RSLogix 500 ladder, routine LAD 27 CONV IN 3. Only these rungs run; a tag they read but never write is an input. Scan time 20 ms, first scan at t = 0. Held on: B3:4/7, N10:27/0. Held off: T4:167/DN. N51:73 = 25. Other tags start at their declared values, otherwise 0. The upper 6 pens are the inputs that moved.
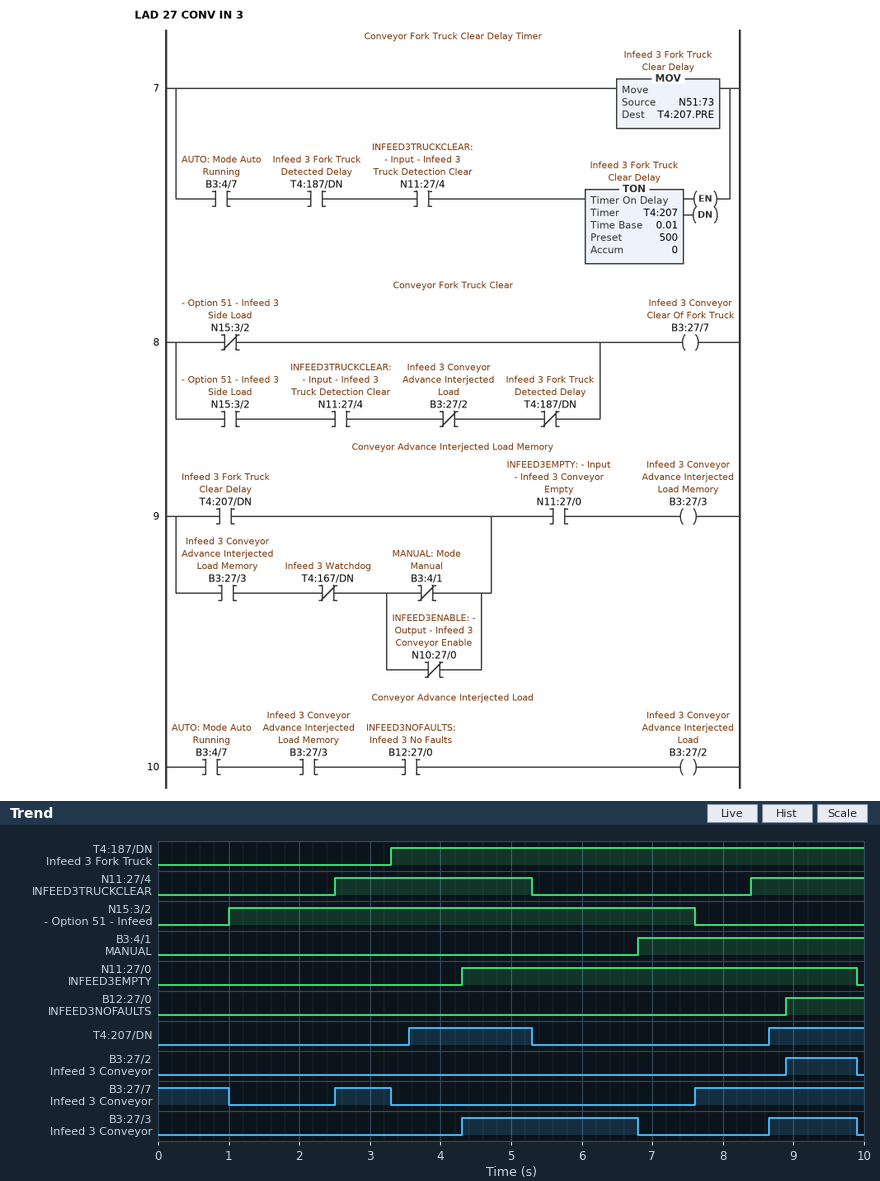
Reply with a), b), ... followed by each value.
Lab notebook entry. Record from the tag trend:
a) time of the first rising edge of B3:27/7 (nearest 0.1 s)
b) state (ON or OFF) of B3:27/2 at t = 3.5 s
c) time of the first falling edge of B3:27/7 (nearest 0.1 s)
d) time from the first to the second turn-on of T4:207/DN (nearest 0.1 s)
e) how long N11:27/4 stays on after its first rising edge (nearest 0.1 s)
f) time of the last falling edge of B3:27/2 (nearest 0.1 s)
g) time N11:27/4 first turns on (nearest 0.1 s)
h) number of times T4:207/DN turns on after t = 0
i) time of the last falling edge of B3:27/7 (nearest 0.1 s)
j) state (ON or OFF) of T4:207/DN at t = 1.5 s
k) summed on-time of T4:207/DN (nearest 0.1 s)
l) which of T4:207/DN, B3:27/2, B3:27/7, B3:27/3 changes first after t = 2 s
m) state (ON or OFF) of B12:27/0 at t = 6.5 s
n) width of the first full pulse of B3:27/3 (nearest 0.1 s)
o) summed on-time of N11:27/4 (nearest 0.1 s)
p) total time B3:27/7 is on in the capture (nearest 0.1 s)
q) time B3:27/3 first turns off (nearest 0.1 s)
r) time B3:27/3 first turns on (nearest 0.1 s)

a) 2.5 s
b) OFF
c) 1.0 s
d) 5.1 s
e) 2.8 s
f) 9.9 s
g) 2.5 s
h) 2
i) 3.3 s
j) OFF
k) 3.1 s
l) B3:27/7
m) OFF
n) 2.5 s
o) 4.4 s
p) 4.2 s
q) 6.8 s
r) 4.3 s
